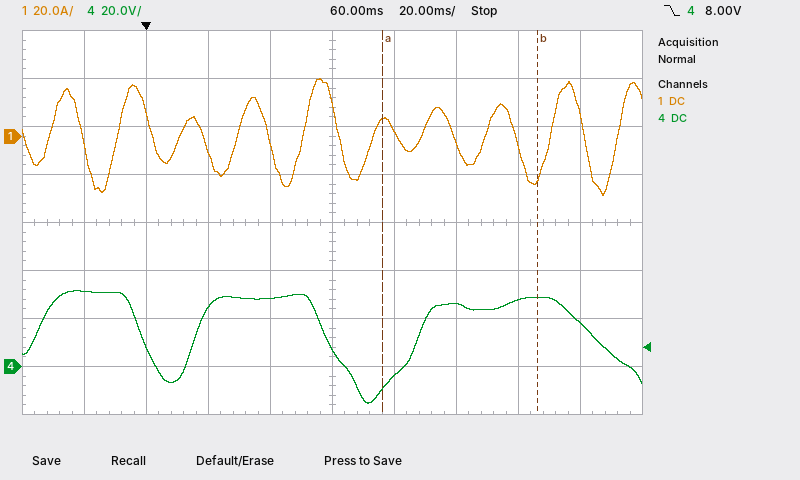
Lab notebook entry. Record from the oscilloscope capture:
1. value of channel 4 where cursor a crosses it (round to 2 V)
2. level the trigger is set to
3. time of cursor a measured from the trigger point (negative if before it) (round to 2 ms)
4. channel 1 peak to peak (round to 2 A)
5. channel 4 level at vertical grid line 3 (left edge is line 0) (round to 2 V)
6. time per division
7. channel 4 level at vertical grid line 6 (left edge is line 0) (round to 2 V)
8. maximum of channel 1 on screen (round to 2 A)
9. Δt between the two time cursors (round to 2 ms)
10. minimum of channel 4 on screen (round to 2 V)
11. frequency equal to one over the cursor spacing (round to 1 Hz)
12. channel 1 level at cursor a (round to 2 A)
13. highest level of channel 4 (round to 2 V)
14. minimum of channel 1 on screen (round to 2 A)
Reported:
-10 V
8.00 V
+76 ms
48 A
24 V
20 ms
-4 V
24 A
50 ms
-16 V
20 Hz
6 A
32 V
-24 A
